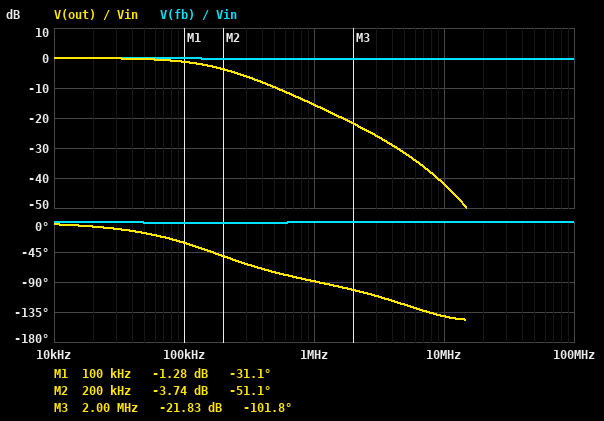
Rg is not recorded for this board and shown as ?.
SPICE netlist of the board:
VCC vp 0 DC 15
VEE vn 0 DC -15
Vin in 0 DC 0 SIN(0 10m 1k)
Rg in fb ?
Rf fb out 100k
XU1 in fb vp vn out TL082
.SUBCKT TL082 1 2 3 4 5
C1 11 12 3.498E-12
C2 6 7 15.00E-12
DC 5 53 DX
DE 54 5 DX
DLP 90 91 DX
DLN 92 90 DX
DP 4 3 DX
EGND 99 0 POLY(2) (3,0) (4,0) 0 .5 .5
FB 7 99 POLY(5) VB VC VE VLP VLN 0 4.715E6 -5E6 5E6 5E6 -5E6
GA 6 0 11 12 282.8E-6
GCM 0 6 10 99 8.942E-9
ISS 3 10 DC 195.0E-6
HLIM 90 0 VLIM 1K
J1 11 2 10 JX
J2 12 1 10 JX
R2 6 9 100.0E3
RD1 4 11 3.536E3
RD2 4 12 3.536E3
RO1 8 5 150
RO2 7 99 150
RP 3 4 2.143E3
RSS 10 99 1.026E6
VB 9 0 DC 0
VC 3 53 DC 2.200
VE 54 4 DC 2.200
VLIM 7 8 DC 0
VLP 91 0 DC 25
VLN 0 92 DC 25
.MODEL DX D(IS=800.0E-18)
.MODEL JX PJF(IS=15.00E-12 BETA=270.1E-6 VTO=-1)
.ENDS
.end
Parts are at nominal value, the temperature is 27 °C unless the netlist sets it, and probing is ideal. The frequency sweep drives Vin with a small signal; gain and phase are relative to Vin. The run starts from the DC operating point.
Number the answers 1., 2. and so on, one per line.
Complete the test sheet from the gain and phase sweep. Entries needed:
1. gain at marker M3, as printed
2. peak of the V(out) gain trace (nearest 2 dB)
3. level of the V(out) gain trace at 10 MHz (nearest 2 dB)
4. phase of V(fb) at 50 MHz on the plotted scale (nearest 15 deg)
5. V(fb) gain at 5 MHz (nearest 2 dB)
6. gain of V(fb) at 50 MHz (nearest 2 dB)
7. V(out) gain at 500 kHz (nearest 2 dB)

1. -21.83 dB
2. 0 dB
3. -42 dB
4. 0 deg
5. 0 dB
6. 0 dB
7. -10 dB
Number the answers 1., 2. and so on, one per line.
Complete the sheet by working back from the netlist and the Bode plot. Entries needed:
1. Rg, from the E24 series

1. 5.1 kΩ
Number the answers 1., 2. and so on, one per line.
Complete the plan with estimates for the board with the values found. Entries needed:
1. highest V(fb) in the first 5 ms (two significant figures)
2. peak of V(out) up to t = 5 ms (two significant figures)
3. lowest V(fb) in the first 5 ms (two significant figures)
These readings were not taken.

1. 10 mV
2. 10 mV
3. -10 mV
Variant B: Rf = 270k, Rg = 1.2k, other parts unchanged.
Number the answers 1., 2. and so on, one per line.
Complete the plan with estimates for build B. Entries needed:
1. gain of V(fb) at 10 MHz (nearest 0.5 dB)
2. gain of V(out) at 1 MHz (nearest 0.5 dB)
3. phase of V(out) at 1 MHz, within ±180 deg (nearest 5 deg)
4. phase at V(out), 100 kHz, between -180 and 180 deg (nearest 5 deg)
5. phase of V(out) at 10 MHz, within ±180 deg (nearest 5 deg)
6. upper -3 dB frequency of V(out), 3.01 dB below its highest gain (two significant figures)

1. 0 dB
2. -36.5 dB
3. -95 deg
4. -80 deg
5. -110 deg
6. 15 kHz
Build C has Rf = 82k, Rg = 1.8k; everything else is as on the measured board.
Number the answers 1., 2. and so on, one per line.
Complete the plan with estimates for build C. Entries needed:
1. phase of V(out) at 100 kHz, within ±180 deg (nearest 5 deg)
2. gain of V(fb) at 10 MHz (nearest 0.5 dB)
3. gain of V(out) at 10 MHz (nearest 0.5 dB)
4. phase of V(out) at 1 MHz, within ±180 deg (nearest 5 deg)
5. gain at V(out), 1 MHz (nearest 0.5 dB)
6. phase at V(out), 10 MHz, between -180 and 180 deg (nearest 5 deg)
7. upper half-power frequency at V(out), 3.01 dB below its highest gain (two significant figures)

1. -55 deg
2. 0 dB
3. -51.5 dB
4. -95 deg
5. -22.5 dB
6. -125 deg
7. 75 kHz
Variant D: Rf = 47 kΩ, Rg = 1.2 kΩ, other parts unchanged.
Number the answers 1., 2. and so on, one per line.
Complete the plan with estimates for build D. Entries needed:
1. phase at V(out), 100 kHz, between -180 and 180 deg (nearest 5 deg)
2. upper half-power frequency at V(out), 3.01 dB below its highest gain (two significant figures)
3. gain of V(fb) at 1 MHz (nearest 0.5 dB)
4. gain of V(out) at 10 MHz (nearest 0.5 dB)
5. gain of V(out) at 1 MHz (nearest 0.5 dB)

1. -50 deg
2. 87 kHz
3. 0 dB
4. -51.5 dB
5. -21.5 dB
